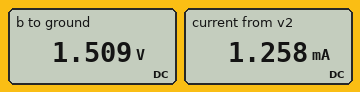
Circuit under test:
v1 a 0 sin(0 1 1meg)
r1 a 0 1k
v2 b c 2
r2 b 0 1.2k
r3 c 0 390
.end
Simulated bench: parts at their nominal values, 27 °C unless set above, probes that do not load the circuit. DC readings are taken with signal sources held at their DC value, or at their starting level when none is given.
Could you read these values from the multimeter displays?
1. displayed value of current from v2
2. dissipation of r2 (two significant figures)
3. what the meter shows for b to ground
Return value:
1.258 mA
1.9 mW
1.509 V
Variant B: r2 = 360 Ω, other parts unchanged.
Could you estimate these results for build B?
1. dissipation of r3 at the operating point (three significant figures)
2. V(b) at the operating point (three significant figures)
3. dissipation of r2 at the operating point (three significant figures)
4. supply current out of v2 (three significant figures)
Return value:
2.77 mW
960 mV
2.56 mW
2.67 mA
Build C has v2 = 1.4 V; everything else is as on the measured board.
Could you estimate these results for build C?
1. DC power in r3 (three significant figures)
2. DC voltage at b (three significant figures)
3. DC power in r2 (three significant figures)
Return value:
302 µW
1.06 V
930 µW
